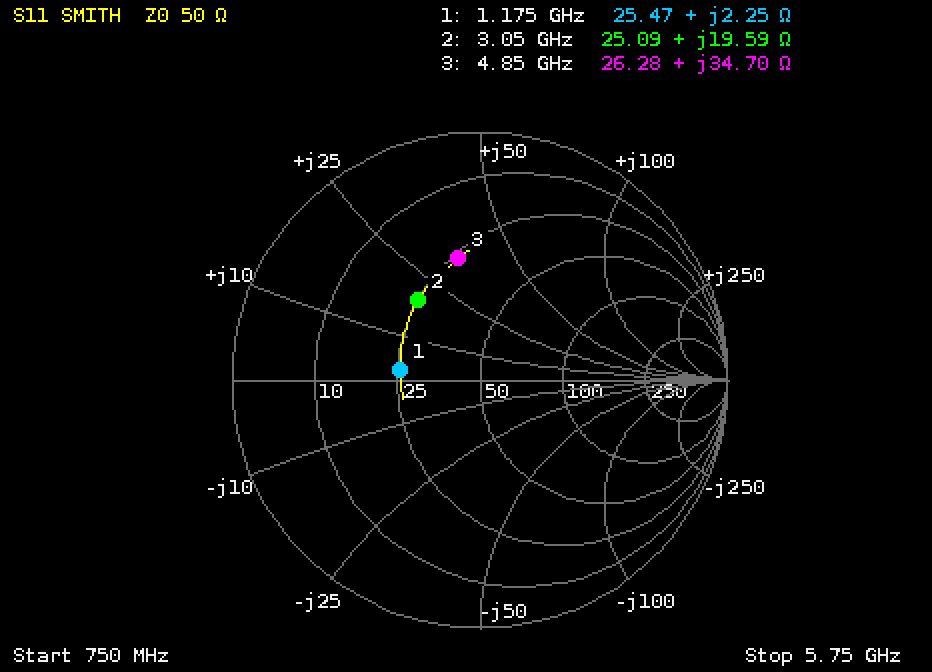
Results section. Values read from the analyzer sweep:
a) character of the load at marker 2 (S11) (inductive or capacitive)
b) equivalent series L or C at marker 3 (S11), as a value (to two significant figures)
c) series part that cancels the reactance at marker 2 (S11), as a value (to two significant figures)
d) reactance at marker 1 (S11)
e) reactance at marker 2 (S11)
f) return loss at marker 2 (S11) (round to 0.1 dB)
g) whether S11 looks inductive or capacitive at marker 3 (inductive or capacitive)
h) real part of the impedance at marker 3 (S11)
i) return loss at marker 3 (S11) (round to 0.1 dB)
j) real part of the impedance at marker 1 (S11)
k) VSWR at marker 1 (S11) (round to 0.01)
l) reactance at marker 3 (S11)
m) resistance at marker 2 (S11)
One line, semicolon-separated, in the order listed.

inductive; 1.1 nH; 2.7 pF; +2.25 Ω; +19.59 Ω; 7.8 dB; inductive; 26.28 Ω; 6.0 dB; 25.47 Ω; 1.97; +34.70 Ω; 25.09 Ω
